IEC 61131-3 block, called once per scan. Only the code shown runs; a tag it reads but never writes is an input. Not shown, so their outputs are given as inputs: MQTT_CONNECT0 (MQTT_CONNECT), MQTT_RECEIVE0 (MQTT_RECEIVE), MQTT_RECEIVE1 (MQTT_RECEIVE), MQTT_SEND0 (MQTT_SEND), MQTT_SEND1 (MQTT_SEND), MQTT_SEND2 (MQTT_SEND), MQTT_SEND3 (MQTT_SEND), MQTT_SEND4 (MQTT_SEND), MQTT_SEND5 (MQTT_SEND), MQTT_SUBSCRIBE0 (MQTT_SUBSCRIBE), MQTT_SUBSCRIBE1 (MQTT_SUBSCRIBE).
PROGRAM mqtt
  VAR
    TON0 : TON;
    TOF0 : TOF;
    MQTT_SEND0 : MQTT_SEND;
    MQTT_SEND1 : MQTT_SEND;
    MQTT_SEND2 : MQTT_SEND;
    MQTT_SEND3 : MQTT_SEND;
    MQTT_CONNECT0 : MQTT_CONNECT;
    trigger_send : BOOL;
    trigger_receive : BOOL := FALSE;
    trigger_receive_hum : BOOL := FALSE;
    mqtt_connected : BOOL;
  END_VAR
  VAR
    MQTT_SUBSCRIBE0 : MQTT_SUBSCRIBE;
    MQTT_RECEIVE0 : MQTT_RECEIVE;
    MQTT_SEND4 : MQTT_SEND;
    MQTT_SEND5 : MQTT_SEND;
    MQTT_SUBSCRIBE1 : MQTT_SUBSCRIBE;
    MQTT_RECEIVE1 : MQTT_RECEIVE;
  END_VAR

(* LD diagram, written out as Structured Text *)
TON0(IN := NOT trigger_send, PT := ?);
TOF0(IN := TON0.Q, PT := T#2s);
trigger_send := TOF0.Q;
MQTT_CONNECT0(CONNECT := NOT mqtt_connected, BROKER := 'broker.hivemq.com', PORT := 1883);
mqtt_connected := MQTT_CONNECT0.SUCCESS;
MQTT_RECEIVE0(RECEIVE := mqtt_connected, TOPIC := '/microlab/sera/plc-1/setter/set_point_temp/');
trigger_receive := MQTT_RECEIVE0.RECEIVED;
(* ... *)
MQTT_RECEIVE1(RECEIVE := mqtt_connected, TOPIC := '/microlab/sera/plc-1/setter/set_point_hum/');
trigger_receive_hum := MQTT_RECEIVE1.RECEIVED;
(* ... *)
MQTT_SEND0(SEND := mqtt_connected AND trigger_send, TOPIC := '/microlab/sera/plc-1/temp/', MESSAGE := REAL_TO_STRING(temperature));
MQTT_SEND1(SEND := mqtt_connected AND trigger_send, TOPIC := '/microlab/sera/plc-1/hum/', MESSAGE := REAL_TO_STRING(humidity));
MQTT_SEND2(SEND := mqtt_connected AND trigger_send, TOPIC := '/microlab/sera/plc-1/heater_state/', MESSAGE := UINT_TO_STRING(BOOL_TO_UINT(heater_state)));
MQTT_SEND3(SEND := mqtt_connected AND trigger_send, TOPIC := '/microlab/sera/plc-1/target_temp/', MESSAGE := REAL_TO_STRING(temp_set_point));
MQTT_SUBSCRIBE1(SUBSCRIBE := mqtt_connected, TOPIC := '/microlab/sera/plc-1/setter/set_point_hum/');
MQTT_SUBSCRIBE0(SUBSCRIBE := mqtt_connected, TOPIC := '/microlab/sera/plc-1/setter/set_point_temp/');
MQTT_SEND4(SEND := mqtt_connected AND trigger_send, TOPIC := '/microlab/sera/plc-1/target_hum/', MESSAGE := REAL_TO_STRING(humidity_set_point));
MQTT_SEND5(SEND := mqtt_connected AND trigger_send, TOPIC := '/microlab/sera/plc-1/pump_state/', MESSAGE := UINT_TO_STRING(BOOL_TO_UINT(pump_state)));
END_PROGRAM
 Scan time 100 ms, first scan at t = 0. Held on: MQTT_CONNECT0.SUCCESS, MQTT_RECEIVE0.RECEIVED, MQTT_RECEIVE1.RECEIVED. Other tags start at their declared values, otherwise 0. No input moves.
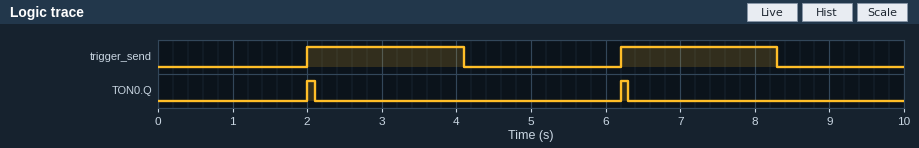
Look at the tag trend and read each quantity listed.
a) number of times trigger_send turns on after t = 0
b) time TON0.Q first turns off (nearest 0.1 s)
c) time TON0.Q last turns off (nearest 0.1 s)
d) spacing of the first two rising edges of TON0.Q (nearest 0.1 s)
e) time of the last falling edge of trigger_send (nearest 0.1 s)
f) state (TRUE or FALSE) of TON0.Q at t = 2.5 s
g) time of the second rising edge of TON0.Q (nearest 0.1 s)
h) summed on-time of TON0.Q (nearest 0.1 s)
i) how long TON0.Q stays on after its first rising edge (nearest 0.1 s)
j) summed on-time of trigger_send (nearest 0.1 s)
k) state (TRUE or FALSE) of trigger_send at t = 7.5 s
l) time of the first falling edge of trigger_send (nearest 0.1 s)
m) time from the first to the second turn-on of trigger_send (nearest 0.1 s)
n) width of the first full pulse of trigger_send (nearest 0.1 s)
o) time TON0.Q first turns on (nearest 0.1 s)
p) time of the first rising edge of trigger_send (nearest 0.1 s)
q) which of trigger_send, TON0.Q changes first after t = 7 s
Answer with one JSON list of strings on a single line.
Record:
["2", "2.1 s", "6.3 s", "4.2 s", "8.3 s", "FALSE", "6.2 s", "0.2 s", "0.1 s", "4.2 s", "TRUE", "4.1 s", "4.2 s", "2.1 s", "2.0 s", "2.0 s", "trigger_send"]
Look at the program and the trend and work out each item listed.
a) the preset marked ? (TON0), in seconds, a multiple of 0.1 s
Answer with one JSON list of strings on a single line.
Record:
["2.0 s"]
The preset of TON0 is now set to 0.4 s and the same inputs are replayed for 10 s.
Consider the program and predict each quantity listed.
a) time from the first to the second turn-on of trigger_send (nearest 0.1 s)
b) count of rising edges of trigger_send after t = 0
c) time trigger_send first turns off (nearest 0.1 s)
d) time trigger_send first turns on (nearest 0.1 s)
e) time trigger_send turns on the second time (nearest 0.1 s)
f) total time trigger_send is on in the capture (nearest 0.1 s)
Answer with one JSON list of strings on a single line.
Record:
["2.6 s", "4", "2.5 s", "0.4 s", "3.0 s", "8.1 s"]
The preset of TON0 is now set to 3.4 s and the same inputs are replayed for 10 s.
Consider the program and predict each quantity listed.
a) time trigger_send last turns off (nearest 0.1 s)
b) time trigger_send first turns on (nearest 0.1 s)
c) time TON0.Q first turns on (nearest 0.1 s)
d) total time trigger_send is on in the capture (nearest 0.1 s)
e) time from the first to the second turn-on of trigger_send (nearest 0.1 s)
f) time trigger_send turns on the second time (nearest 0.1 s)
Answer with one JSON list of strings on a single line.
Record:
["5.5 s", "3.4 s", "3.4 s", "3.1 s", "5.6 s", "9.0 s"]
